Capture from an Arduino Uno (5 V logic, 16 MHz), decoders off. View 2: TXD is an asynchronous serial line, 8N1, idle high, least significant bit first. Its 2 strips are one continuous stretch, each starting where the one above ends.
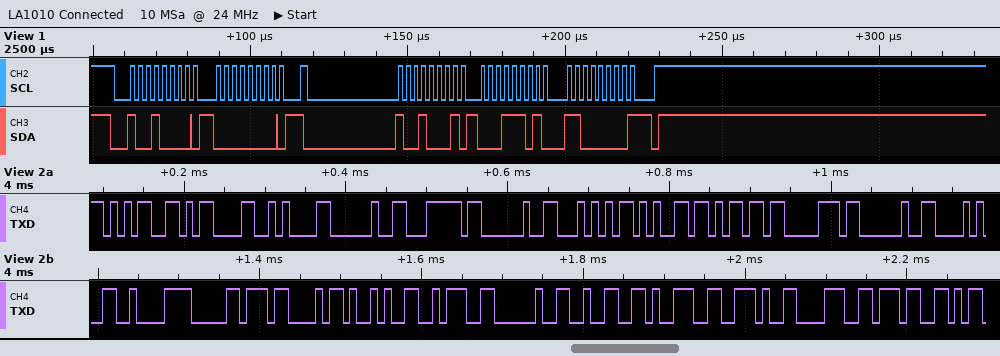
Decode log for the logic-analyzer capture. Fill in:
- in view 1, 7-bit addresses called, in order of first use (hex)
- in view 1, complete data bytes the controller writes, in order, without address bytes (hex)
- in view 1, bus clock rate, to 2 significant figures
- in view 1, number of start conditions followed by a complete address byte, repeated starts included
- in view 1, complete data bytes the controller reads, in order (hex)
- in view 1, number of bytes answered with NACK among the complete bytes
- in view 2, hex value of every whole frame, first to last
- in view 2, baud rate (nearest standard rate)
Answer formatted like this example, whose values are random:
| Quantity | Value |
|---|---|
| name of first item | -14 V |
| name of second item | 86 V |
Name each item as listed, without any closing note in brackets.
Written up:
| Quantity | Value |
|---|---|
| in view 1, 7-bit addresses called, in order of first use | 0x48 |
| in view 1, complete data bytes the controller writes, in order, without address bytes | 00 |
| in view 1, bus clock rate, to 2 significant figures | 400 kHz |
| in view 1, number of start conditions followed by a complete address byte, repeated starts included | 2 |
| in view 1, complete data bytes the controller reads, in order | 1D C0 |
| in view 1, number of bytes answered with NACK among the complete bytes | 1 |
| in view 2, hex value of every whole frame, first to last | 35 0D 0A 20 7C 20 54 65 6D 70 20 28 C2 B0 43 29 3A 20 32 39 2E 38 37 |
| in view 2, baud rate | 115200 baud |
